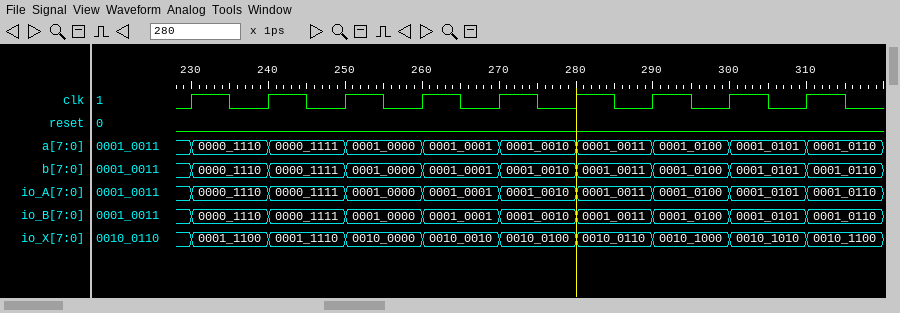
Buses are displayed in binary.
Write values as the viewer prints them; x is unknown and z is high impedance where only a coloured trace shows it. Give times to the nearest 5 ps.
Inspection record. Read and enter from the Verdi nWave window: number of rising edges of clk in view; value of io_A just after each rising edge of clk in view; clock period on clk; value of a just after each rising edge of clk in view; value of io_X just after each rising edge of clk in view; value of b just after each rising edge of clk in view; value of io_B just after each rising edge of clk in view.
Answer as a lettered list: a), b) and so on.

a) 9
b) 0000_1110, 0000_1111, 0001_0000, 0001_0001, 0001_0010, 0001_0011, 0001_0100, 0001_0101, 0001_0110
c) 10 ps
d) 0000_1110, 0000_1111, 0001_0000, 0001_0001, 0001_0010, 0001_0011, 0001_0100, 0001_0101, 0001_0110
e) 0001_1100, 0001_1110, 0010_0000, 0010_0010, 0010_0100, 0010_0110, 0010_1000, 0010_1010, 0010_1100
f) 0000_1110, 0000_1111, 0001_0000, 0001_0001, 0001_0010, 0001_0011, 0001_0100, 0001_0101, 0001_0110
g) 0000_1110, 0000_1111, 0001_0000, 0001_0001, 0001_0010, 0001_0011, 0001_0100, 0001_0101, 0001_0110
